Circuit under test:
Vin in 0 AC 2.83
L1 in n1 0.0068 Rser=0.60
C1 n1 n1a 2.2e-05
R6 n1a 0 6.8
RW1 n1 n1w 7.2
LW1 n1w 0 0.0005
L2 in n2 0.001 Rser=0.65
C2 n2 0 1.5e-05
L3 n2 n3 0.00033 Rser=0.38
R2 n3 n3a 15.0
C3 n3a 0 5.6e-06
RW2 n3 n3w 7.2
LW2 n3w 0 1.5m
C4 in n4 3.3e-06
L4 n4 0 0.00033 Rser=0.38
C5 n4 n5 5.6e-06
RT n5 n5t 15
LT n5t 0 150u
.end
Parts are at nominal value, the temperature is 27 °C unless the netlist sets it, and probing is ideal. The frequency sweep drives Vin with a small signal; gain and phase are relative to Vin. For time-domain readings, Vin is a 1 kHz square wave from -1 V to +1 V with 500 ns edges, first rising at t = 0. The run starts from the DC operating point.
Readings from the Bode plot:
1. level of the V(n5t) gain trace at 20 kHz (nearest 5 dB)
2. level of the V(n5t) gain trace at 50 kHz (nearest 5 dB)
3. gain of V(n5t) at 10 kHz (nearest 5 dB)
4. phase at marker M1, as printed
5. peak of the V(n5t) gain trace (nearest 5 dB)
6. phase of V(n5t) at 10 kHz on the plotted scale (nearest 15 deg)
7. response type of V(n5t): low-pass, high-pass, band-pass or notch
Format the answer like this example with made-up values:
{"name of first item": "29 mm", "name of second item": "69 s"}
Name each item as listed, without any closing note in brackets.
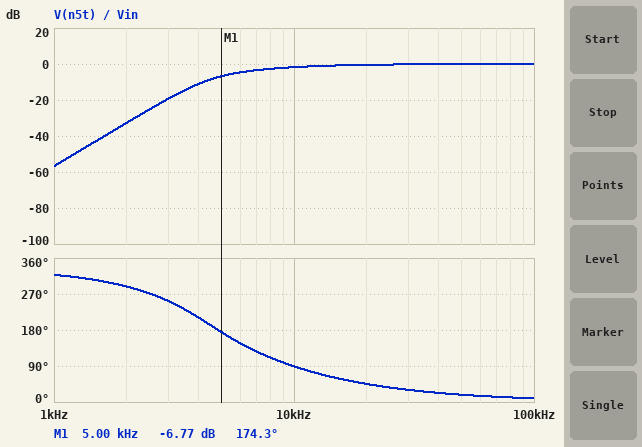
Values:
{"level of the V(n5t) gain trace at 20 kHz": "0 dB", "level of the V(n5t) gain trace at 50 kHz": "0 dB", "gain of V(n5t) at 10 kHz": "0 dB", "phase at marker M1, as printed": "174.3 deg", "peak of the V(n5t) gain trace": "0 dB", "phase of V(n5t) at 10 kHz on the plotted scale": "90 deg", "response type of V(n5t): low-pass, high-pass, band-pass or notch": "high-pass"}
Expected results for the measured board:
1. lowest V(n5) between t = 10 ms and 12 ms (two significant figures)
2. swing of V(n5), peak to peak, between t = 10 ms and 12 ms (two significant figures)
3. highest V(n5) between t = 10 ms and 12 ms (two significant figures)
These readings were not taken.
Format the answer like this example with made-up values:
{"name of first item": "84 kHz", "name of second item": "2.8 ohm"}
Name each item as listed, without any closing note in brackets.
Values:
{"lowest V(n5) between t = 10 ms and 12 ms": "-2.0 V", "swing of V(n5), peak to peak, between t = 10 ms and 12 ms": "4.0 V", "highest V(n5) between t = 10 ms and 12 ms": "2.0 V"}
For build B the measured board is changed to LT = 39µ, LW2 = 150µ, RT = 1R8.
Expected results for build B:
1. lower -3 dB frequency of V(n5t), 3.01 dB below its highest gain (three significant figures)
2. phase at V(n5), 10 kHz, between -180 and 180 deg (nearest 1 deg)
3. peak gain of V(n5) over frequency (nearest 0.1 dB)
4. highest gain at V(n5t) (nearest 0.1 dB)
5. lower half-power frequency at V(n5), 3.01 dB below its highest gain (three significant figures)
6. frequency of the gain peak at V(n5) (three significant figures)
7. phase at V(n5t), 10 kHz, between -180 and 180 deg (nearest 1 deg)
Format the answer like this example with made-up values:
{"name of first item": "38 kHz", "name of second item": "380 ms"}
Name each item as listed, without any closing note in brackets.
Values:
{"lower -3 dB frequency of V(n5t), 3.01 dB below its highest gain": "15.7 kHz", "phase at V(n5), 10 kHz, between -180 and 180 deg": "129 deg", "peak gain of V(n5) over frequency": "9.2 dB", "highest gain at V(n5t)": "8.6 dB", "lower half-power frequency at V(n5), 3.01 dB below its highest gain": "15.6 kHz", "frequency of the gain peak at V(n5)": "18.6 kHz", "phase at V(n5t), 10 kHz, between -180 and 180 deg": "165 deg"}
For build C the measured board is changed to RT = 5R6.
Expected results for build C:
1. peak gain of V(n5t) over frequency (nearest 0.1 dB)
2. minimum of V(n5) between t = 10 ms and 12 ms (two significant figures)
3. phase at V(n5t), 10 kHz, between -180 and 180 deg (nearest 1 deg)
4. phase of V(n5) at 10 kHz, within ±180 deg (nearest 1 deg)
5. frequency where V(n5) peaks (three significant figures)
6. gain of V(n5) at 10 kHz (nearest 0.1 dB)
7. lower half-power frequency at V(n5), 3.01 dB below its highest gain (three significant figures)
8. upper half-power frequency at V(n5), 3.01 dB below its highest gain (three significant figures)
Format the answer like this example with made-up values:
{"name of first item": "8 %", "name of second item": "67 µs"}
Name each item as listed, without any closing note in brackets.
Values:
{"peak gain of V(n5t) over frequency": "6.8 dB", "minimum of V(n5) between t = 10 ms and 12 ms": "-2.0 V", "phase at V(n5t), 10 kHz, between -180 and 180 deg": "87 deg", "phase of V(n5) at 10 kHz, within ±180 deg": "57 deg", "frequency where V(n5) peaks": "9.97 kHz", "gain of V(n5) at 10 kHz": "8.1 dB", "lower half-power frequency at V(n5), 3.01 dB below its highest gain": "7.87 kHz", "upper half-power frequency at V(n5), 3.01 dB below its highest gain": "13.9 kHz"}
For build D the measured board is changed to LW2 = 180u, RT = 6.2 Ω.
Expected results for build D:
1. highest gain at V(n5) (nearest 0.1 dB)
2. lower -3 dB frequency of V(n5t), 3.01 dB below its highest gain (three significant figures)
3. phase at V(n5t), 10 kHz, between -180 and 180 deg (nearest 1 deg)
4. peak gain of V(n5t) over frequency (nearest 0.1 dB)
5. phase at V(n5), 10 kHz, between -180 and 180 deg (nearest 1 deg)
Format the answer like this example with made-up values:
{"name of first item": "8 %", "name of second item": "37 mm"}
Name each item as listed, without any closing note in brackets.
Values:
{"highest gain at V(n5)": "7.4 dB", "lower -3 dB frequency of V(n5t), 3.01 dB below its highest gain": "7.95 kHz", "phase at V(n5t), 10 kHz, between -180 and 180 deg": "88 deg", "peak gain of V(n5t) over frequency": "5.9 dB", "phase at V(n5), 10 kHz, between -180 and 180 deg": "54 deg"}
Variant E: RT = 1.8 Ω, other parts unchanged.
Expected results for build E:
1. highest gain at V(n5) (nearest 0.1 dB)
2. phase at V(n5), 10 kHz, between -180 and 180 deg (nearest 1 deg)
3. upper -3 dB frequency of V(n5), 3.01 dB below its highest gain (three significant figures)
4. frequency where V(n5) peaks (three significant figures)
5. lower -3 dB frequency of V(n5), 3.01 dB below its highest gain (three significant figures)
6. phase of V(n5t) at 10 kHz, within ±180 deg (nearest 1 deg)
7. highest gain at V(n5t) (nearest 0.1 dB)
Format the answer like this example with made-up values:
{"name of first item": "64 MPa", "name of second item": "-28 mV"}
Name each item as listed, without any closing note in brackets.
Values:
{"highest gain at V(n5)": "16.6 dB", "phase at V(n5), 10 kHz, between -180 and 180 deg": "70 deg", "upper -3 dB frequency of V(n5), 3.01 dB below its highest gain": "10.8 kHz", "frequency where V(n5) peaks": "9.90 kHz", "lower -3 dB frequency of V(n5), 3.01 dB below its highest gain": "9.16 kHz", "phase of V(n5t) at 10 kHz, within ±180 deg": "81 deg", "highest gain at V(n5t)": "16.5 dB"}
